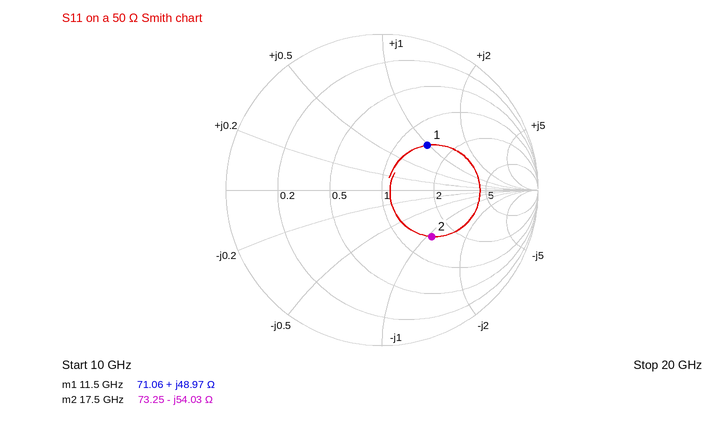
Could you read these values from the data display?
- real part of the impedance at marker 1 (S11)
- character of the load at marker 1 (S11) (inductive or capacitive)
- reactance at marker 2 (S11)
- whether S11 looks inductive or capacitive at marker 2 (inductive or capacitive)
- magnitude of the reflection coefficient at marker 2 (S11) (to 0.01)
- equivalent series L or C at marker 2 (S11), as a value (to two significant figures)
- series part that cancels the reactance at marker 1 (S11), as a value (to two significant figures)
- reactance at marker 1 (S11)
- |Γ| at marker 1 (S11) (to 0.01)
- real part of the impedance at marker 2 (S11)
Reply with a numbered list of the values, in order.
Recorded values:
1. 71.06 Ω
2. inductive
3. -54.03 Ω
4. capacitive
5. 0.44
6. 170 fF
7. 280 fF
8. +48.97 Ω
9. 0.41
10. 73.25 Ω
